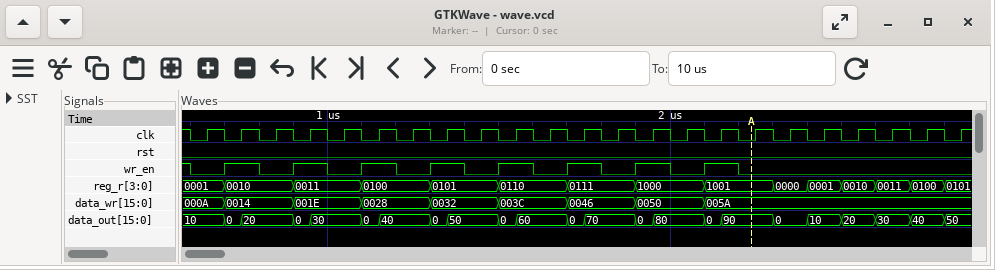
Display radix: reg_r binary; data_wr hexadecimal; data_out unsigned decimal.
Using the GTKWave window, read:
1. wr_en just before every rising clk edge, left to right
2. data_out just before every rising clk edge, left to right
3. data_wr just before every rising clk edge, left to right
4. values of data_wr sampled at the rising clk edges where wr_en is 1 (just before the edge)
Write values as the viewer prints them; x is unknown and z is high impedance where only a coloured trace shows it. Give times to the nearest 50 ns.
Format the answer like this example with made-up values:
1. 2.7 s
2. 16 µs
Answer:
1. 0 1 0 1 0 1 0 1 0 1 0 1 0 1 0 1 0 0 0 0 0 0 0
2. 10, 0, 20, 0, 30, 0, 40, 0, 50, 0, 60, 0, 70, 0, 80, 0, 90, 0, 10, 20, 30, 40, 50
3. 000A, 0014, 0014, 001E, 001E, 0028, 0028, 0032, 0032, 003C, 003C, 0046, 0046, 0050, 0050, 005A, 005A, 005A, 005A, 005A, 005A, 005A, 005A
4. 0014, 001E, 0028, 0032, 003C, 0046, 0050, 005A
